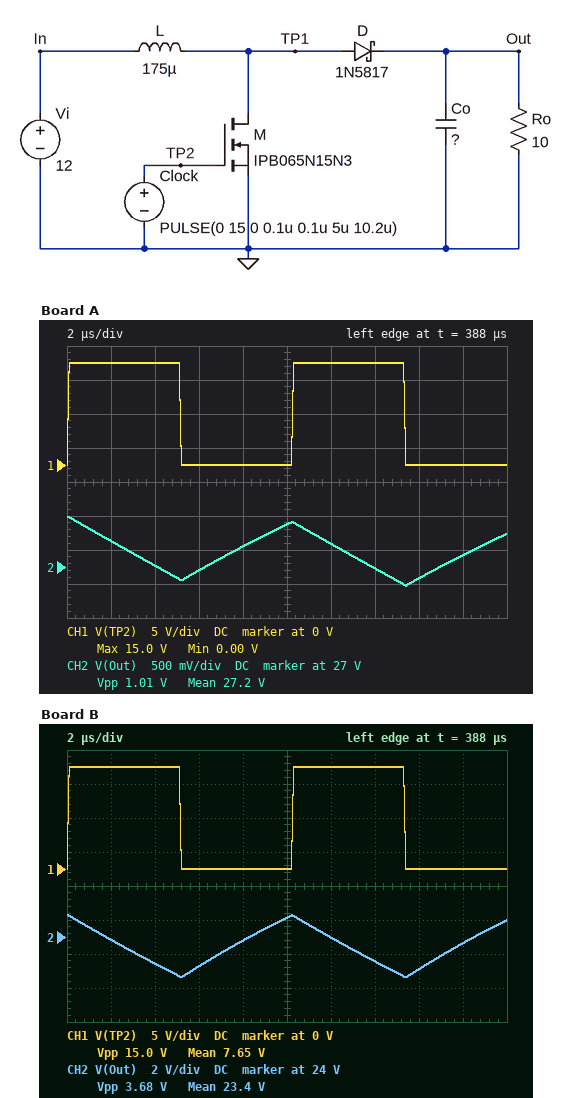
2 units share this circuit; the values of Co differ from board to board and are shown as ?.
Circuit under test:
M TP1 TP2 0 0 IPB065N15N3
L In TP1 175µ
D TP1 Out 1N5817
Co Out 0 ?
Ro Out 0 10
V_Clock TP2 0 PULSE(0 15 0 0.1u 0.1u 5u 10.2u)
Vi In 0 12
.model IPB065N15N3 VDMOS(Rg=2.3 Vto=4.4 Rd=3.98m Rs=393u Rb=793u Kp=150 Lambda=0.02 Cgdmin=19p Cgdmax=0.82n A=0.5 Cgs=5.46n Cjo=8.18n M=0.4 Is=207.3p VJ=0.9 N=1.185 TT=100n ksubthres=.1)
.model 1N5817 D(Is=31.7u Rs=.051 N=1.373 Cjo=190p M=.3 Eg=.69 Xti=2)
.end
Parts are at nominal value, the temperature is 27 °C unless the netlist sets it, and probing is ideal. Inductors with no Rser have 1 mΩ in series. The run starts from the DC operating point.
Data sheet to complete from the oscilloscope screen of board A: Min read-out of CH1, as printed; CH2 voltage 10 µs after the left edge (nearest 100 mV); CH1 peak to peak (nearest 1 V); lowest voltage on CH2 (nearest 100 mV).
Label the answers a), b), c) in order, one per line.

a) 0.00 V
b) 27.6 V
c) 15 V
d) 26.7 V
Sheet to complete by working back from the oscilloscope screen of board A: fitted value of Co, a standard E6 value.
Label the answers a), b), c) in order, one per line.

a) 15 µF
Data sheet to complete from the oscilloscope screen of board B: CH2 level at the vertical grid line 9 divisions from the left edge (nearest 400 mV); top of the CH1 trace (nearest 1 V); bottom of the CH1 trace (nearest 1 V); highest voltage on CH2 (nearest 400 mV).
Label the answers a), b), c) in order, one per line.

a) 23.6 V
b) 15 V
c) 0 V
d) 25.2 V
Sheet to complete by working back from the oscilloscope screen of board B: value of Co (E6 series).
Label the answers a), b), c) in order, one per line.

a) 3.3 µF
